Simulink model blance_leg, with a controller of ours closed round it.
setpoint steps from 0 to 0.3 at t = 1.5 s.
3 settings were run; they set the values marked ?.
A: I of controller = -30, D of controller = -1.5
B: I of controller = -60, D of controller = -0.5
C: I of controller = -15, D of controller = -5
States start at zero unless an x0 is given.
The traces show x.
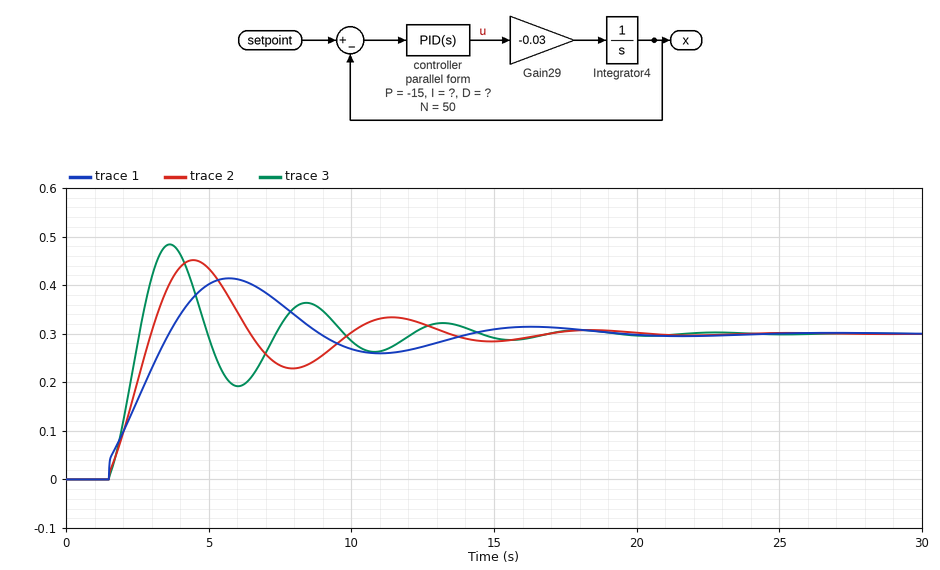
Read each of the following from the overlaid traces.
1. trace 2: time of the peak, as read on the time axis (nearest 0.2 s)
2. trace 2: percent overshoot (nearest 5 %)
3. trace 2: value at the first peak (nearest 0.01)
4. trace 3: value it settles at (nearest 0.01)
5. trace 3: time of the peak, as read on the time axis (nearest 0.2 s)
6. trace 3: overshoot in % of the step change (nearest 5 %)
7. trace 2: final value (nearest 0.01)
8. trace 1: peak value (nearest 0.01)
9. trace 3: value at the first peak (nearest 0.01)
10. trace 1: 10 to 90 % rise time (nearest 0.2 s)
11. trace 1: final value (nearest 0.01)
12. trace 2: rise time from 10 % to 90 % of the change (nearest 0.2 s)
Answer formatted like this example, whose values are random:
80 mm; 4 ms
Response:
4.4 s; 50 %; 0.45; 0.30; 3.6 s; 60 %; 0.30; 0.41; 0.48; 1.8 s; 0.30; 1.2 s
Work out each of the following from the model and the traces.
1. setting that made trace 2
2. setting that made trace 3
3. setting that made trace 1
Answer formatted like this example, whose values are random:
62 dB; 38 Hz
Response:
A; B; C
